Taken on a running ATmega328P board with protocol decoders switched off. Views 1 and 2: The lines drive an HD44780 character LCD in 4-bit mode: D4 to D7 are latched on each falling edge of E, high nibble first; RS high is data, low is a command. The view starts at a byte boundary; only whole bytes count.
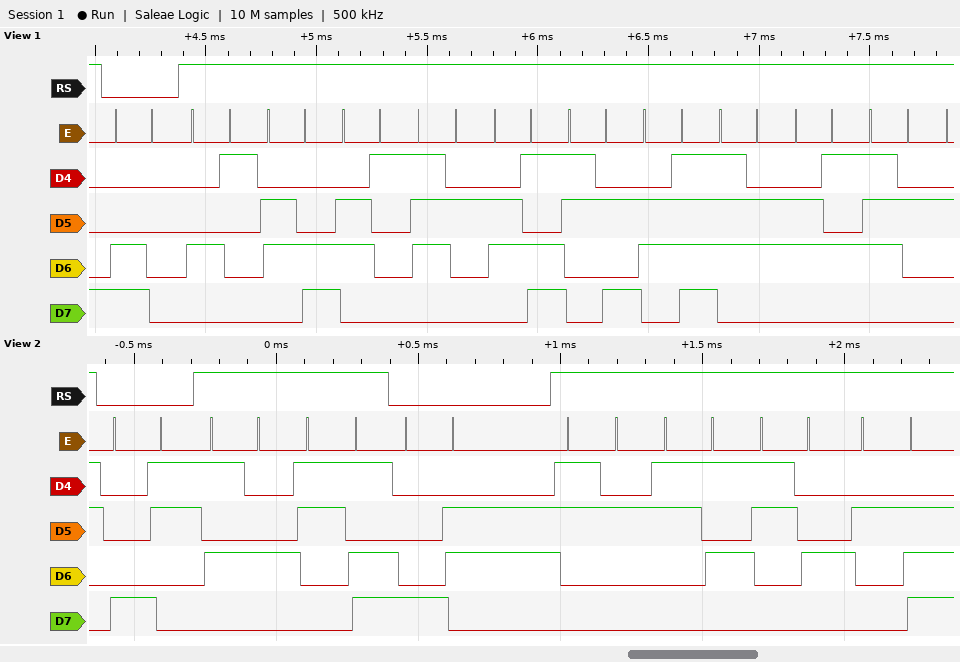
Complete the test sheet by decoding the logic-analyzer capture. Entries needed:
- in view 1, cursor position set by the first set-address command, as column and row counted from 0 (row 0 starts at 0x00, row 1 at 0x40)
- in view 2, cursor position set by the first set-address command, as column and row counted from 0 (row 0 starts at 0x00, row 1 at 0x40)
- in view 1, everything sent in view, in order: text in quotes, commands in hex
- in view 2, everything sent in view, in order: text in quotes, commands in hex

column 0, row 1
column 3, row 0
0xC0 "Alarm:over"
0x83 "T=" 0x86 "254."
